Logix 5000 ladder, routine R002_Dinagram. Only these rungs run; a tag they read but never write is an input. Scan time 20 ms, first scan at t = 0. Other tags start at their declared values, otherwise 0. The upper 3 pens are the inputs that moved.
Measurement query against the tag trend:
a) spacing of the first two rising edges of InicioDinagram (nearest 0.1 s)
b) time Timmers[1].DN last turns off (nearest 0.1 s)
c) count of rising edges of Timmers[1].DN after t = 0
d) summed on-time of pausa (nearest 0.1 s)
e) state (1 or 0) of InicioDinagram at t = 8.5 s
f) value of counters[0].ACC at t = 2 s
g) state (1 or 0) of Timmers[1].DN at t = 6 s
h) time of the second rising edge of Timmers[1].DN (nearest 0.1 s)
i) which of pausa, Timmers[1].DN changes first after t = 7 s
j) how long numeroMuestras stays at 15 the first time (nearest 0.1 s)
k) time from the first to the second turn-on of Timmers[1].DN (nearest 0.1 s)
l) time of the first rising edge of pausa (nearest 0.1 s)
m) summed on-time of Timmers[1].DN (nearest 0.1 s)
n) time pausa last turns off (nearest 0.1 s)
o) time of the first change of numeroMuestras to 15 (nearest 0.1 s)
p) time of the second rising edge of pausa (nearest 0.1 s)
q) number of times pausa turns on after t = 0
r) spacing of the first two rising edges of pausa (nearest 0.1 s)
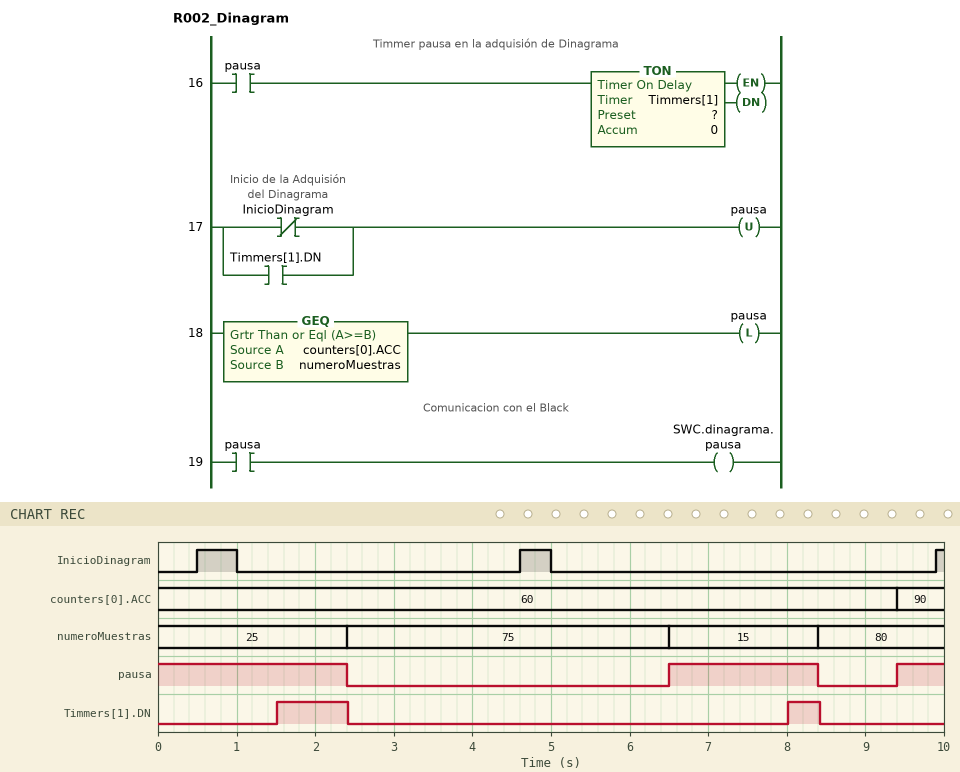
4.1 s
8.4 s
2
4.9 s
0
60
0
8.0 s
Timmers[1].DN
1.9 s
6.5 s
6.5 s
1.3 s
8.4 s
6.5 s
9.4 s
2
2.9 s
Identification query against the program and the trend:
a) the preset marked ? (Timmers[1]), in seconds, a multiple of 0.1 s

1.5 s
